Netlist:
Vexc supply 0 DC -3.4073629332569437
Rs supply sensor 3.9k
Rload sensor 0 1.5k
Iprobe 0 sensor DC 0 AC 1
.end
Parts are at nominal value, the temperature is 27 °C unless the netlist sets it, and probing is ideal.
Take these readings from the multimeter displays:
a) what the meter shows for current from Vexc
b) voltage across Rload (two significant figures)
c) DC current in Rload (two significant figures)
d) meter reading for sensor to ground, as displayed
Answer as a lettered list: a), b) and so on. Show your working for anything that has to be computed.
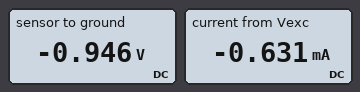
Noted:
a) -0.631 mA
b) 0 V - (-946 mV) = 950 mV
c) (0 V - (-946 mV)) / 1.5 kΩ = 630 µA
d) -0.946 V
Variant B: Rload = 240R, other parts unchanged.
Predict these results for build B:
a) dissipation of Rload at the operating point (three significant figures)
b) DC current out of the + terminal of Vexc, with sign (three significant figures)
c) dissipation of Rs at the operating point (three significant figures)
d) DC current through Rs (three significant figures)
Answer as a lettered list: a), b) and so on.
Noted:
a) 163 µW
b) -823 µA
c) 2.64 mW
d) 823 µA
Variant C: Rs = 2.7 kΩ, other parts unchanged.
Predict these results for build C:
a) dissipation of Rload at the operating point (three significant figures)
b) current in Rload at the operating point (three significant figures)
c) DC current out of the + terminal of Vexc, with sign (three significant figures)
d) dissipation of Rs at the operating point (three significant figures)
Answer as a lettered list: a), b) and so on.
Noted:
a) 987 µW
b) 811 µA
c) -811 µA
d) 1.78 mW
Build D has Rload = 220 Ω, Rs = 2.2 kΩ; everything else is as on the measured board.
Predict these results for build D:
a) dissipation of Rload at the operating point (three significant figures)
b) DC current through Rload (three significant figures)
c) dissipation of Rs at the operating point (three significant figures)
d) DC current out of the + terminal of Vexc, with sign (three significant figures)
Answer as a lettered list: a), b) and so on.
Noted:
a) 436 µW
b) 1.41 mA
c) 4.36 mW
d) -1.41 mA
